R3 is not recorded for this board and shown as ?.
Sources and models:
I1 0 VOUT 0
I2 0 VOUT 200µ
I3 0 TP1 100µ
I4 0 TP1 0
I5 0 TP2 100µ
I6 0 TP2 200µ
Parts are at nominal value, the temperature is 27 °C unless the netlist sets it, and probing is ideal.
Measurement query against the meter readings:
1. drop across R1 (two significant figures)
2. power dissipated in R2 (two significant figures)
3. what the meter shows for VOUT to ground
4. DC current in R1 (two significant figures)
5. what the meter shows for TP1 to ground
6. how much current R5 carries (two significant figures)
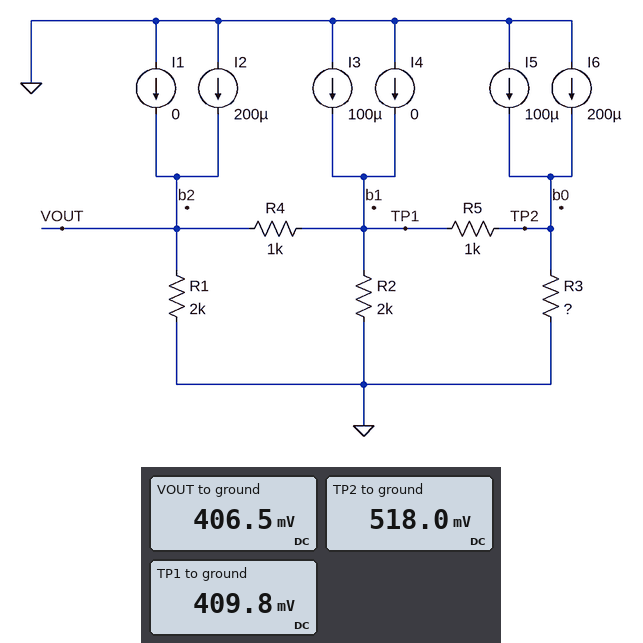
410 mV
84 µW
406.5 mV
200 µA
409.8 mV
110 µA
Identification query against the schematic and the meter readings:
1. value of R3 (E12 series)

2.7 kΩ
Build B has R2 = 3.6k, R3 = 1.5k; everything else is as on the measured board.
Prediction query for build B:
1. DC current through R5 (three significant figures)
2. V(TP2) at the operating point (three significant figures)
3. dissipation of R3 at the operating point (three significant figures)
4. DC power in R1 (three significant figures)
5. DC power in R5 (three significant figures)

16.5 µA
425 mV
121 µW
82.4 µW
272 nW
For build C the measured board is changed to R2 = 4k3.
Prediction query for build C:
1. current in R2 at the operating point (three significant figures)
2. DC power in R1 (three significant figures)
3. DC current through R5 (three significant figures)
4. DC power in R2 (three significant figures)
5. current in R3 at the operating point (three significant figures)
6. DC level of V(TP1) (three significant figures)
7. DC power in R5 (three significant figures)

126 µA
122 µW
72.7 µA
68.0 µW
227 µA
541 mV
5.29 µW
